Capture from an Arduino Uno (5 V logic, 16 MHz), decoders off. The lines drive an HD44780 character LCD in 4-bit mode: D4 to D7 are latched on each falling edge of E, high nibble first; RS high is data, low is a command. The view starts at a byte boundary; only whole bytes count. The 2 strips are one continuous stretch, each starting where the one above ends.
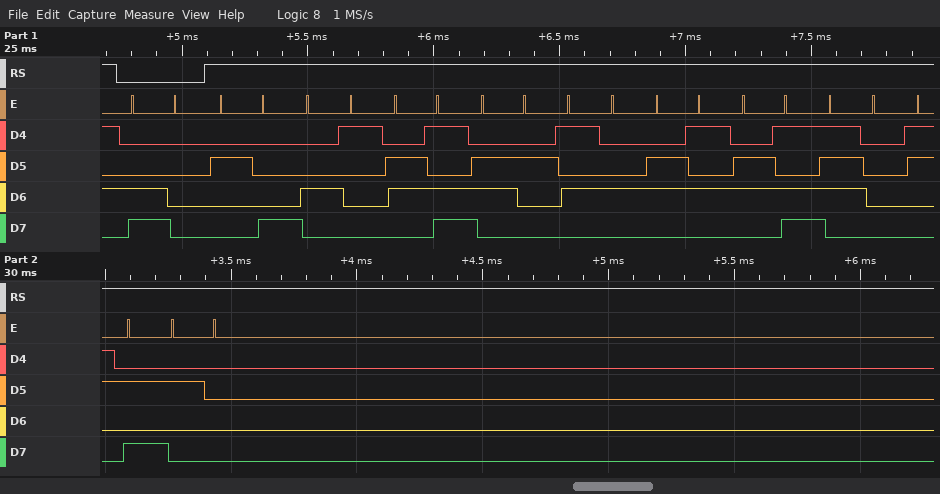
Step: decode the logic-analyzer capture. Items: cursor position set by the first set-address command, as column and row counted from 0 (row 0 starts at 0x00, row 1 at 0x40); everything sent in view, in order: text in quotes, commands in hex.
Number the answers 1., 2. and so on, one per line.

1. column 0, row 1
2. 0xC0 "(AmbTemp: "
